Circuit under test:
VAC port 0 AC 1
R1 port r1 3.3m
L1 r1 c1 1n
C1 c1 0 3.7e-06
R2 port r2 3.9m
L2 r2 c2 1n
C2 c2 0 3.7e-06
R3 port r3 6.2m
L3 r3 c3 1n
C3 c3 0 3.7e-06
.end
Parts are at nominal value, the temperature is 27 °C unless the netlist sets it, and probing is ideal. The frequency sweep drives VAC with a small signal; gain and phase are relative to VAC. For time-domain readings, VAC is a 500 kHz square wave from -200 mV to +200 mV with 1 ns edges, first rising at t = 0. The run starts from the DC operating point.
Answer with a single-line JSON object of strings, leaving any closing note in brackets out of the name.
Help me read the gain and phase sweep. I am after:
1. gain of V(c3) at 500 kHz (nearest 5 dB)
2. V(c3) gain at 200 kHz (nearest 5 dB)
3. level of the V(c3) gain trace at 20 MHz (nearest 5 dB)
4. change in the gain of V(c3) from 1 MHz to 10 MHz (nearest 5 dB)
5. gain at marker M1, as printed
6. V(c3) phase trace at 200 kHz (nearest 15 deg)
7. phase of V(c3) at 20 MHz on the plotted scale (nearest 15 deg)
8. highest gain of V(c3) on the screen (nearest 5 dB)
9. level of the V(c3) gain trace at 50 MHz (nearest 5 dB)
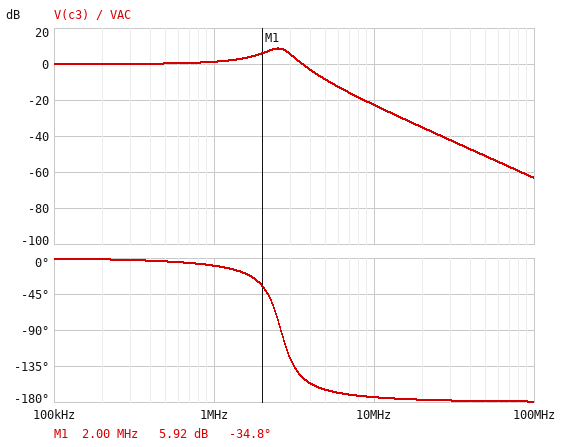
{"gain of V(c3) at 500 kHz": "0 dB", "V(c3) gain at 200 kHz": "0 dB", "level of the V(c3) gain trace at 20 MHz": "-35 dB", "change in the gain of V(c3) from 1 MHz to 10 MHz": "-25 dB", "gain at marker M1, as printed": "5.92 dB", "V(c3) phase trace at 200 kHz": "0 deg", "phase of V(c3) at 20 MHz on the plotted scale": "-180 deg", "highest gain of V(c3) on the screen": "10 dB", "level of the V(c3) gain trace at 50 MHz": "-50 dB"}
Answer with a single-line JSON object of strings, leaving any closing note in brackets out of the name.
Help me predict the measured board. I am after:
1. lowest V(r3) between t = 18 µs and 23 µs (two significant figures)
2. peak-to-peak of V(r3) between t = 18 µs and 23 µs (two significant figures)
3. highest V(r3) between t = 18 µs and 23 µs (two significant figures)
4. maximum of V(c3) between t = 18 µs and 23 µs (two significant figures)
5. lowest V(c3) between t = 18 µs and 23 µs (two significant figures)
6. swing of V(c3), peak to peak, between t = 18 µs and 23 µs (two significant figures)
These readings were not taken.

{"lowest V(r3) between t = 18 µs and 23 µs": "-270 mV", "peak-to-peak of V(r3) between t = 18 µs and 23 µs": "530 mV", "highest V(r3) between t = 18 µs and 23 µs": "270 mV", "maximum of V(c3) between t = 18 µs and 23 µs": "430 mV", "lowest V(c3) between t = 18 µs and 23 µs": "-430 mV", "swing of V(c3), peak to peak, between t = 18 µs and 23 µs": "860 mV"}
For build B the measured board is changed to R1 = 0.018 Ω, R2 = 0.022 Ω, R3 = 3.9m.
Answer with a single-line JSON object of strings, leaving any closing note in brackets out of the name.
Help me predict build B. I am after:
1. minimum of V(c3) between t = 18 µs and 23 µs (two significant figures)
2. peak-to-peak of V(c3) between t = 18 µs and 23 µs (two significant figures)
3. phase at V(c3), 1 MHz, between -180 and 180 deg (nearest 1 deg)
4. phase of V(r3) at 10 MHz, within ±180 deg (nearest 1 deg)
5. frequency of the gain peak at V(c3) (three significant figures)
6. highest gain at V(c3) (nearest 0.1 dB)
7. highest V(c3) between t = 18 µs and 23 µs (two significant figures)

{"minimum of V(c3) between t = 18 µs and 23 µs": "-510 mV", "peak-to-peak of V(c3) between t = 18 µs and 23 µs": "1.0 V", "phase at V(c3), 1 MHz, between -180 and 180 deg": "-6 deg", "phase of V(r3) at 10 MHz, within ±180 deg": "4 deg", "frequency of the gain peak at V(c3)": "2.58 MHz", "highest gain at V(c3)": "12.6 dB", "highest V(c3) between t = 18 µs and 23 µs": "510 mV"}
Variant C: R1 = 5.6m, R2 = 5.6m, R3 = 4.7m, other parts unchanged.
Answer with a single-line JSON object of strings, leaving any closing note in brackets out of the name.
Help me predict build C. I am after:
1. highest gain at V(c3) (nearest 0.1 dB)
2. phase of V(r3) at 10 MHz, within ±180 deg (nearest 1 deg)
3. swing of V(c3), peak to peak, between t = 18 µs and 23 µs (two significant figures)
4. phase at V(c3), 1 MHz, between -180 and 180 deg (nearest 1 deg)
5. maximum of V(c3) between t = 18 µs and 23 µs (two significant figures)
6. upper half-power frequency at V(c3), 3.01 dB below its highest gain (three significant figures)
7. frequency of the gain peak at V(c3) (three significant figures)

{"highest gain at V(c3)": "11.0 dB", "phase of V(r3) at 10 MHz, within ±180 deg": "5 deg", "swing of V(c3), peak to peak, between t = 18 µs and 23 µs": "960 mV", "phase at V(c3), 1 MHz, between -180 and 180 deg": "-7 deg", "maximum of V(c3) between t = 18 µs and 23 µs": "480 mV", "upper half-power frequency at V(c3), 3.01 dB below its highest gain": "2.92 MHz", "frequency of the gain peak at V(c3)": "2.56 MHz"}
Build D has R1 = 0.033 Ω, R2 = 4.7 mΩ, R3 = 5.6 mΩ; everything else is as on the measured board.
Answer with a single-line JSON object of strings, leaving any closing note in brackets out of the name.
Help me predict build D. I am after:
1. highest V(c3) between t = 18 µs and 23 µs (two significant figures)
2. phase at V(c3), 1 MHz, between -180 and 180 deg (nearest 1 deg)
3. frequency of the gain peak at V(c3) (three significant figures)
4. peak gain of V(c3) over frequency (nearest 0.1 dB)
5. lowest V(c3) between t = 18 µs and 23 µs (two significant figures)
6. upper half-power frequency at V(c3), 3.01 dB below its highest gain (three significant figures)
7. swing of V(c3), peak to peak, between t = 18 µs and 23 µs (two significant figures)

{"highest V(c3) between t = 18 µs and 23 µs": "450 mV", "phase at V(c3), 1 MHz, between -180 and 180 deg": "-9 deg", "frequency of the gain peak at V(c3)": "2.54 MHz", "peak gain of V(c3) over frequency": "9.5 dB", "lowest V(c3) between t = 18 µs and 23 µs": "-450 mV", "upper half-power frequency at V(c3), 3.01 dB below its highest gain": "2.96 MHz", "swing of V(c3), peak to peak, between t = 18 µs and 23 µs": "890 mV"}
